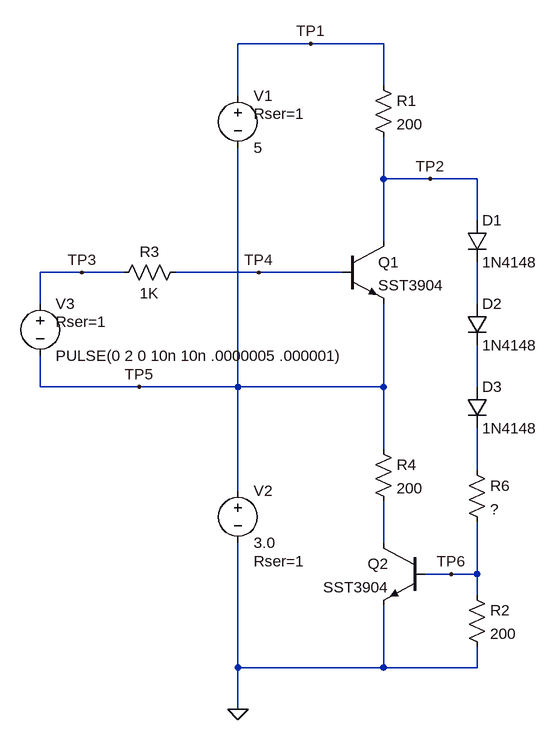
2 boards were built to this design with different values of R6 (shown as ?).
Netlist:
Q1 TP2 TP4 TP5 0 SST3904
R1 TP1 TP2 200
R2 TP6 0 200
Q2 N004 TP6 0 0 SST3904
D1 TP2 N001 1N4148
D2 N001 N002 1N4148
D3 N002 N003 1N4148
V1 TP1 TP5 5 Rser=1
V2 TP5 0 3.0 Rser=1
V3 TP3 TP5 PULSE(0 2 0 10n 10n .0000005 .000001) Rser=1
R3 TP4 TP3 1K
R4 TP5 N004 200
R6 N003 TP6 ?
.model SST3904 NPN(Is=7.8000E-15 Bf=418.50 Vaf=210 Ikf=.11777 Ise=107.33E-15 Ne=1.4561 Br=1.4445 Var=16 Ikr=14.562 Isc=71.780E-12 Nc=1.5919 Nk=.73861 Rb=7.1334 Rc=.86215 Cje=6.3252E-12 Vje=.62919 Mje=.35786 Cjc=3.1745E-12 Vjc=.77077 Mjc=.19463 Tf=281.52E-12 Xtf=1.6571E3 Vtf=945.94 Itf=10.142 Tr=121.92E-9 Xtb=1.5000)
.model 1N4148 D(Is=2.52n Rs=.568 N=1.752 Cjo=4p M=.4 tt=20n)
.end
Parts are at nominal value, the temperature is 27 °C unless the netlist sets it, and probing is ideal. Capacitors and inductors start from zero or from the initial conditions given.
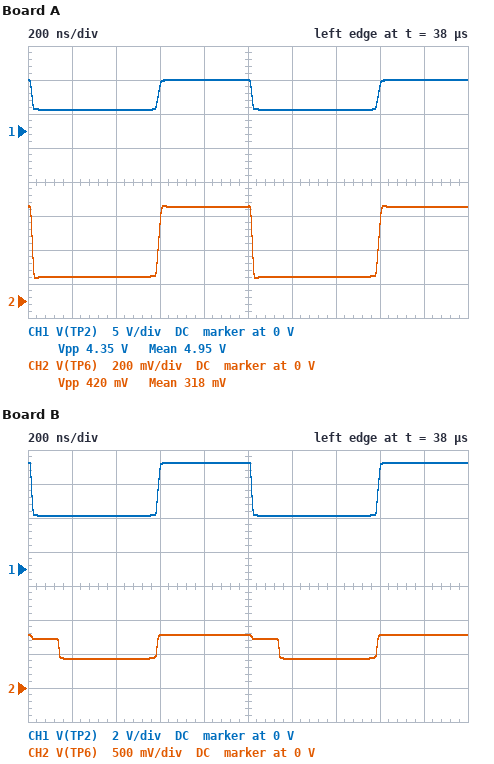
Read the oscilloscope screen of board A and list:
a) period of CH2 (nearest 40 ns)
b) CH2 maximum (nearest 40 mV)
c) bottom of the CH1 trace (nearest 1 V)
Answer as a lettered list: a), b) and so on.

a) 1.00 µs
b) 560 mV
c) 3 V
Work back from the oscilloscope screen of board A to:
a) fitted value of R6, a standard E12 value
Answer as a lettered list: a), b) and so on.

a) 1.8 kΩ
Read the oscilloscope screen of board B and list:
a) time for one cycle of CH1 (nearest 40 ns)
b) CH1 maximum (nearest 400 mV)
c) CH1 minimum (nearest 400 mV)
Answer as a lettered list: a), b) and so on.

a) 1.00 µs
b) 6.4 V
c) 3.2 V
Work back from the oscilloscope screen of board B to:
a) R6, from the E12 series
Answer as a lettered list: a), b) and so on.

a) 390 Ω
